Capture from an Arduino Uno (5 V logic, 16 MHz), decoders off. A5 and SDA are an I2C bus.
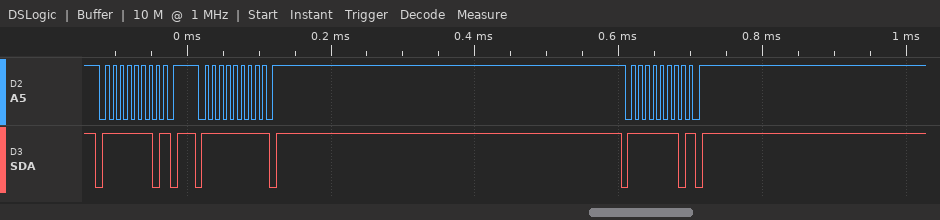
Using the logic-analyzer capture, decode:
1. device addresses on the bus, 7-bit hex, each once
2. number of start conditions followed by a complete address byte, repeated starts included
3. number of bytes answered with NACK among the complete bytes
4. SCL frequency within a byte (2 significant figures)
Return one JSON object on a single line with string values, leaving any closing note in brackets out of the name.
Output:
{"device addresses on the bus, 7-bit hex, each once": "0x7F", "number of start conditions followed by a complete address byte, repeated starts included": "3", "number of bytes answered with NACK among the complete bytes": "3", "SCL frequency within a byte": "100 kHz"}
